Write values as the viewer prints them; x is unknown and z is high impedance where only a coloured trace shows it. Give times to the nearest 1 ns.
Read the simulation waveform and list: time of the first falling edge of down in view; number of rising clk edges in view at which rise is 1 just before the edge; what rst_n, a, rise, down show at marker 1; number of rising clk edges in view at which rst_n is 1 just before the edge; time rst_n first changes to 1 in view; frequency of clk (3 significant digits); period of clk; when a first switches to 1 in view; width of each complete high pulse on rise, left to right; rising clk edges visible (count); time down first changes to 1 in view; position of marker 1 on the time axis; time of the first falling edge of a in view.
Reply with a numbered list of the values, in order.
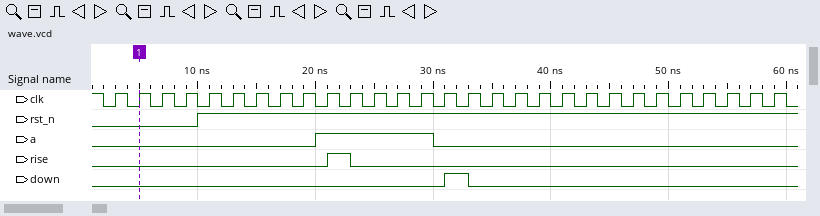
1. 33 ns
2. 1
3. rst_n=0, a=0, rise=0, down=0
4. 25
5. 10 ns
6. 500 MHz
7. 2 ns
8. 20 ns
9. 2 ns
10. 29
11. 31 ns
12. 5 ns
13. 30 ns
